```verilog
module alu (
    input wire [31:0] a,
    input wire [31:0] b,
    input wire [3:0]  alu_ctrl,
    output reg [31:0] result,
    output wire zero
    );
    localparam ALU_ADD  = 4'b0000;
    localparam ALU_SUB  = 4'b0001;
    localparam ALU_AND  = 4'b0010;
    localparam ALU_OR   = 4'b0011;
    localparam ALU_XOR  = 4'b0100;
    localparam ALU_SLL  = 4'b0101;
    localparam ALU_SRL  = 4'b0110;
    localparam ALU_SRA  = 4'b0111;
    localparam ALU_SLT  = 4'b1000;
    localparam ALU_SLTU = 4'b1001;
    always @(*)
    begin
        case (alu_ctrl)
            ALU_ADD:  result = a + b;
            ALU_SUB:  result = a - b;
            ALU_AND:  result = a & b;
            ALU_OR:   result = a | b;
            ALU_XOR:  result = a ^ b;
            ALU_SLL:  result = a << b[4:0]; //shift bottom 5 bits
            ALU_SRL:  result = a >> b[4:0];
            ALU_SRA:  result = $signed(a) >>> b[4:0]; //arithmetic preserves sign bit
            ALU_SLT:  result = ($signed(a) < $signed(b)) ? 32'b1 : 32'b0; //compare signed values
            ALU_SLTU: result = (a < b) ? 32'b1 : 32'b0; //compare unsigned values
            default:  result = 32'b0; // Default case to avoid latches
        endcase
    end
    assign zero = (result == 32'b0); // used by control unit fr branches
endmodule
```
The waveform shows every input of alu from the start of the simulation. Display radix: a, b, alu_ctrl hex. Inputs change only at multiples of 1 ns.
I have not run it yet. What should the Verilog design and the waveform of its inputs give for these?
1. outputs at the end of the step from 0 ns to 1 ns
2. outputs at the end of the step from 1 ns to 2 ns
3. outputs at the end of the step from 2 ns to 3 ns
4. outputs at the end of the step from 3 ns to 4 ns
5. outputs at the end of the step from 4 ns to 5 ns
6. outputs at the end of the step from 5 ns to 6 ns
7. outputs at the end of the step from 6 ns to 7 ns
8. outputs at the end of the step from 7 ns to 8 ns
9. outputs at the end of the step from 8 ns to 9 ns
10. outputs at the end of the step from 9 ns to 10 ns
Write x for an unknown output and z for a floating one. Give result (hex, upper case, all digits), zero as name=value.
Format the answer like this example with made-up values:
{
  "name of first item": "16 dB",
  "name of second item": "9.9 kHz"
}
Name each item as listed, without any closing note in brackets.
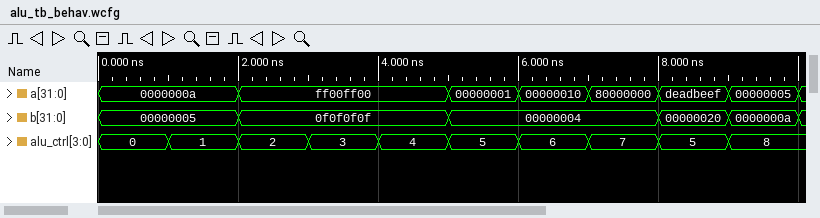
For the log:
{
  "outputs at the end of the step from 0 ns to 1 ns": "result=0000000F, zero=0",
  "outputs at the end of the step from 1 ns to 2 ns": "result=00000005, zero=0",
  "outputs at the end of the step from 2 ns to 3 ns": "result=0F000F00, zero=0",
  "outputs at the end of the step from 3 ns to 4 ns": "result=FF0FFF0F, zero=0",
  "outputs at the end of the step from 4 ns to 5 ns": "result=F00FF00F, zero=0",
  "outputs at the end of the step from 5 ns to 6 ns": "result=00000010, zero=0",
  "outputs at the end of the step from 6 ns to 7 ns": "result=00000001, zero=0",
  "outputs at the end of the step from 7 ns to 8 ns": "result=F8000000, zero=0",
  "outputs at the end of the step from 8 ns to 9 ns": "result=DEADBEEF, zero=0",
  "outputs at the end of the step from 9 ns to 10 ns": "result=00000001, zero=0"
}
